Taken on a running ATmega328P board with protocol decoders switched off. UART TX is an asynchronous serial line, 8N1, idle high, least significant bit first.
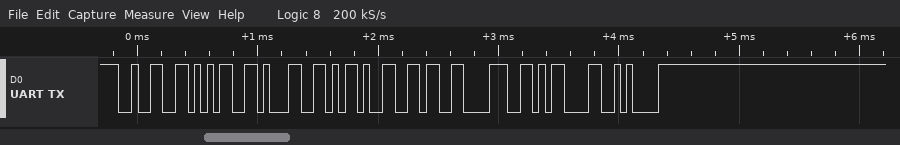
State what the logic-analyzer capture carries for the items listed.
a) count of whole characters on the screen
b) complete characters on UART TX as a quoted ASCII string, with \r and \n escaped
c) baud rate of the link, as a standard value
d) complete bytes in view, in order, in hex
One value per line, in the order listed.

8
"251-68\r\n"
19200 baud
0x32 0x35 0x31 0x2D 0x36 0x38 0x0D 0x0A
